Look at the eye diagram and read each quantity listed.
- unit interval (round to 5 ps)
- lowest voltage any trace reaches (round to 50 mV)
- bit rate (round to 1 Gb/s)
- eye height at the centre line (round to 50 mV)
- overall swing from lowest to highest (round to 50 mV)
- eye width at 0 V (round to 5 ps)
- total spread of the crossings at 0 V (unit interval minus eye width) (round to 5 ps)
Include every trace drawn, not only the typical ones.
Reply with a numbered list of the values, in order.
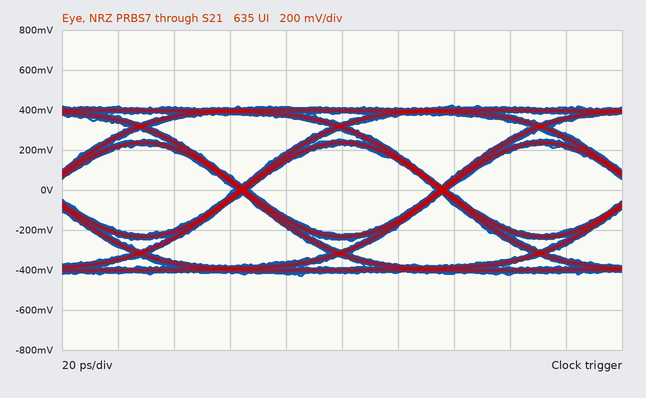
1. 70 ps
2. -450 mV
3. 14 Gb/s
4. 450 mV
5. 850 mV
6. 65 ps
7. 5 ps
